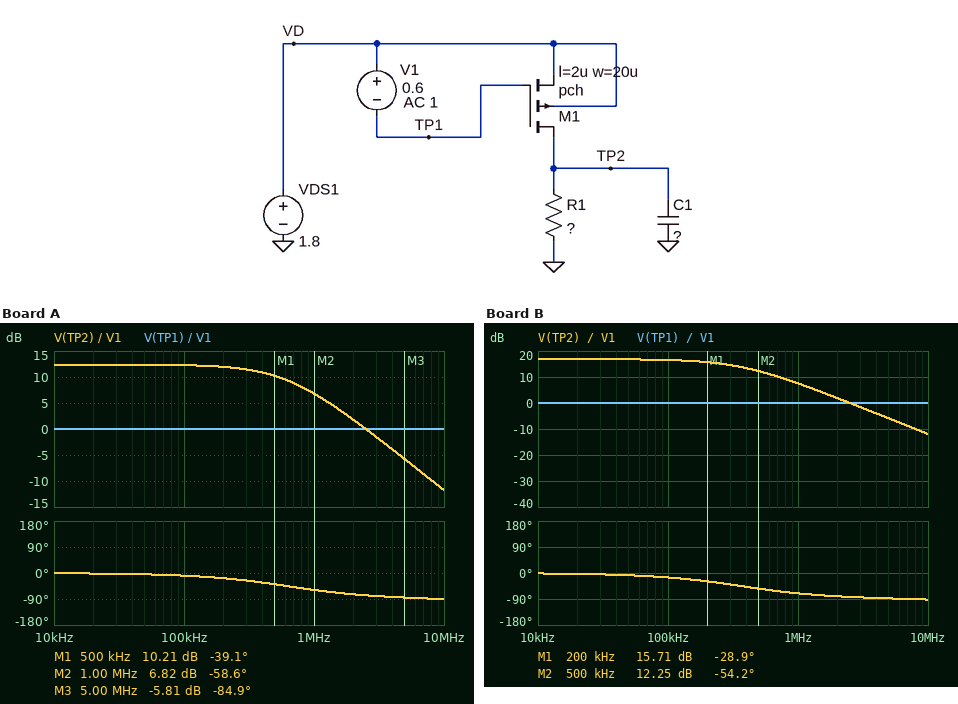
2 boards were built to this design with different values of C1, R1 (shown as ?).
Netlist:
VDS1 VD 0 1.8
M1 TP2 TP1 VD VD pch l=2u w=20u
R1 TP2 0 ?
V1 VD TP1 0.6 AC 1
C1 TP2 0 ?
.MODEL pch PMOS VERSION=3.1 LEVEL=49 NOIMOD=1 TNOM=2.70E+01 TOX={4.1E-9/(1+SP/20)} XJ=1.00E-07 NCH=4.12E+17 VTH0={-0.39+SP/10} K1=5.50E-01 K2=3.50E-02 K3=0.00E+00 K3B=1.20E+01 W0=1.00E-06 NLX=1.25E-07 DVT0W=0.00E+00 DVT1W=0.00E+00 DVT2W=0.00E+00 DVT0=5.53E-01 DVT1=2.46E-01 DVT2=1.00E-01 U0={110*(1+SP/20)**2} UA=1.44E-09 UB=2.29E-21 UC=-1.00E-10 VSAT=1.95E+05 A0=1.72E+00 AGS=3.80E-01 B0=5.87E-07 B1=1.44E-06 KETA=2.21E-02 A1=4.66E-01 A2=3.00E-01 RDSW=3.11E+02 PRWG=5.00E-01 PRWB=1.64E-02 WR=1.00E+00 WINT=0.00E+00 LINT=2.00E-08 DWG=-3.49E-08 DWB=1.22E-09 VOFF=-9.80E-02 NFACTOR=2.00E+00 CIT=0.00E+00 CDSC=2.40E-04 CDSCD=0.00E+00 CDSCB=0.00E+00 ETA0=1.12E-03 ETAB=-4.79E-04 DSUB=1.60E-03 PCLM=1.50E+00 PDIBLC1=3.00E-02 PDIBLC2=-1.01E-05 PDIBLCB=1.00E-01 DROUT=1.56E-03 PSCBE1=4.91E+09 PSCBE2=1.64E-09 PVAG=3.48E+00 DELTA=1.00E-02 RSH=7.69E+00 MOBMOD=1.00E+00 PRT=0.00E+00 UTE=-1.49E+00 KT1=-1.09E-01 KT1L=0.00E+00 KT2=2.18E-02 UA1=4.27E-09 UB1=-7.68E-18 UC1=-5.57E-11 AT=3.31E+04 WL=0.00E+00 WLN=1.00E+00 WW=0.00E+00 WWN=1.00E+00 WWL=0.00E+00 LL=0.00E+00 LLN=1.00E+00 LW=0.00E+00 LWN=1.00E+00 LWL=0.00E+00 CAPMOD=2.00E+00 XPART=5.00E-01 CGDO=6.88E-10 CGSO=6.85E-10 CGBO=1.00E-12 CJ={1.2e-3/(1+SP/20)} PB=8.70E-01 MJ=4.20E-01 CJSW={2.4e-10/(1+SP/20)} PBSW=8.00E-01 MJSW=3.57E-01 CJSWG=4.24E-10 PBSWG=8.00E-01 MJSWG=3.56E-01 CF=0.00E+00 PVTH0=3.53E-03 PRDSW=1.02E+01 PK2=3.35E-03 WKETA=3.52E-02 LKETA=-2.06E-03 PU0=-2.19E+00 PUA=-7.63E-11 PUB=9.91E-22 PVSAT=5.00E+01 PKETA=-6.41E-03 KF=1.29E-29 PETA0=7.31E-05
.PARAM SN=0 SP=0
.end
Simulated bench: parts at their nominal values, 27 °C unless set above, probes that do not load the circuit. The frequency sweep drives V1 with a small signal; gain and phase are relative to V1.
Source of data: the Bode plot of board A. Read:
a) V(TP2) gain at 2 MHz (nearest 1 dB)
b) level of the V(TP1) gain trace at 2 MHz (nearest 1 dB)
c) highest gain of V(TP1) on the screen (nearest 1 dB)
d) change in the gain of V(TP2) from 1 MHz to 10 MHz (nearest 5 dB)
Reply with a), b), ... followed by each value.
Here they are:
a) 2 dB
b) 0 dB
c) 0 dB
d) -20 dB
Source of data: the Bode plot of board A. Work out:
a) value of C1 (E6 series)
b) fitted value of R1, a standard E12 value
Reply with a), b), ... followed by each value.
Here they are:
a) 6.8 pF
b) 39 kΩ
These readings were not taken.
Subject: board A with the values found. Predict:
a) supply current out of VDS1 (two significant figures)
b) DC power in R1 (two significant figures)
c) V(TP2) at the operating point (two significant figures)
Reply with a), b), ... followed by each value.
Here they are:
a) 12 µA
b) 5.4 µW
c) 460 mV
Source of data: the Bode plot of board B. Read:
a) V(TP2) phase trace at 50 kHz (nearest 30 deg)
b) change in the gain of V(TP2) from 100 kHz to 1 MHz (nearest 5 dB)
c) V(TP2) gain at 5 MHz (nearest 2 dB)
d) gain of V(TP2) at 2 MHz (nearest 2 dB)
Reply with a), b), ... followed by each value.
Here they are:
a) 0 deg
b) -10 dB
c) -6 dB
d) 2 dB
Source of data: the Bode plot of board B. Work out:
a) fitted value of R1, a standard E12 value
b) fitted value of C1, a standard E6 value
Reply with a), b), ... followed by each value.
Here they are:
a) 68 kΩ
b) 6.8 pF
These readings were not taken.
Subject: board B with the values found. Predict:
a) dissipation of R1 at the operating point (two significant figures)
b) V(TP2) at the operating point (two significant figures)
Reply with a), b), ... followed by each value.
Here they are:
a) 8.9 µW
b) 780 mV
